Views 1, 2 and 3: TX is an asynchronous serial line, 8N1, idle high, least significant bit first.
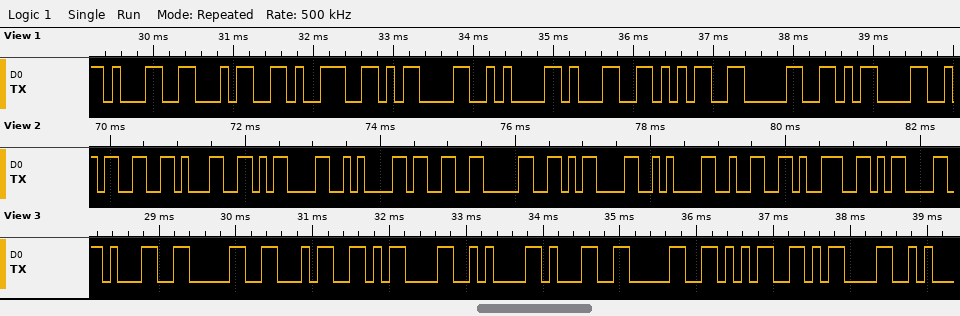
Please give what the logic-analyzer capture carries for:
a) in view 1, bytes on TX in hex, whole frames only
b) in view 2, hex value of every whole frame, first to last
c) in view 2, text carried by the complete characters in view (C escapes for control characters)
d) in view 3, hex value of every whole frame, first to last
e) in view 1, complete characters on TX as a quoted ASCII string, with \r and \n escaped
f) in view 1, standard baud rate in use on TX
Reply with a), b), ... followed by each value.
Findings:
a) 31 34 39 0D 0A 31 35 30 0D
b) 0x33 0x31 0x0D 0x0A 0x33 0x30 0x0D 0x0A 0x32 0x39 0x0D
c) "31\r\n30\r\n29\r"
d) 31 30 34 0D 0A 31 30 35 0D
e) "149\r\n150\r"
f) 9600 baud
